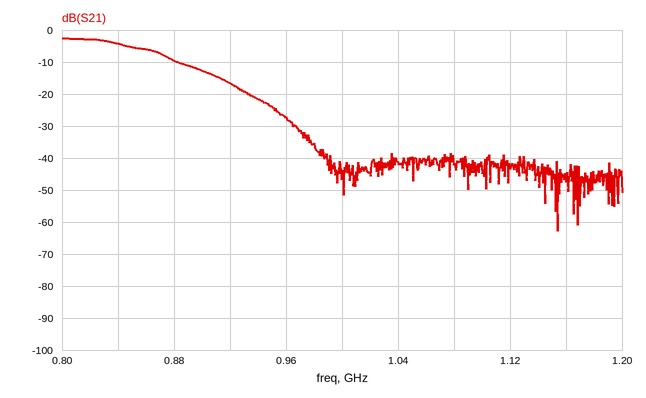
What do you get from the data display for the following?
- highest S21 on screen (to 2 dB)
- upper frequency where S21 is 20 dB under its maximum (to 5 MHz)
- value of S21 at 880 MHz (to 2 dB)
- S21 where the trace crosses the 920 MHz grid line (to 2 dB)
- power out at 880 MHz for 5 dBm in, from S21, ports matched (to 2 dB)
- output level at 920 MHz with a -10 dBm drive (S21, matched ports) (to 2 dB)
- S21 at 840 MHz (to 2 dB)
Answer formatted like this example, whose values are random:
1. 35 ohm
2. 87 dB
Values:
1. -2 dB
2. 945 MHz
3. -10 dB
4. -16 dB
5. -4 dBm
6. -26 dBm
7. -4 dB
